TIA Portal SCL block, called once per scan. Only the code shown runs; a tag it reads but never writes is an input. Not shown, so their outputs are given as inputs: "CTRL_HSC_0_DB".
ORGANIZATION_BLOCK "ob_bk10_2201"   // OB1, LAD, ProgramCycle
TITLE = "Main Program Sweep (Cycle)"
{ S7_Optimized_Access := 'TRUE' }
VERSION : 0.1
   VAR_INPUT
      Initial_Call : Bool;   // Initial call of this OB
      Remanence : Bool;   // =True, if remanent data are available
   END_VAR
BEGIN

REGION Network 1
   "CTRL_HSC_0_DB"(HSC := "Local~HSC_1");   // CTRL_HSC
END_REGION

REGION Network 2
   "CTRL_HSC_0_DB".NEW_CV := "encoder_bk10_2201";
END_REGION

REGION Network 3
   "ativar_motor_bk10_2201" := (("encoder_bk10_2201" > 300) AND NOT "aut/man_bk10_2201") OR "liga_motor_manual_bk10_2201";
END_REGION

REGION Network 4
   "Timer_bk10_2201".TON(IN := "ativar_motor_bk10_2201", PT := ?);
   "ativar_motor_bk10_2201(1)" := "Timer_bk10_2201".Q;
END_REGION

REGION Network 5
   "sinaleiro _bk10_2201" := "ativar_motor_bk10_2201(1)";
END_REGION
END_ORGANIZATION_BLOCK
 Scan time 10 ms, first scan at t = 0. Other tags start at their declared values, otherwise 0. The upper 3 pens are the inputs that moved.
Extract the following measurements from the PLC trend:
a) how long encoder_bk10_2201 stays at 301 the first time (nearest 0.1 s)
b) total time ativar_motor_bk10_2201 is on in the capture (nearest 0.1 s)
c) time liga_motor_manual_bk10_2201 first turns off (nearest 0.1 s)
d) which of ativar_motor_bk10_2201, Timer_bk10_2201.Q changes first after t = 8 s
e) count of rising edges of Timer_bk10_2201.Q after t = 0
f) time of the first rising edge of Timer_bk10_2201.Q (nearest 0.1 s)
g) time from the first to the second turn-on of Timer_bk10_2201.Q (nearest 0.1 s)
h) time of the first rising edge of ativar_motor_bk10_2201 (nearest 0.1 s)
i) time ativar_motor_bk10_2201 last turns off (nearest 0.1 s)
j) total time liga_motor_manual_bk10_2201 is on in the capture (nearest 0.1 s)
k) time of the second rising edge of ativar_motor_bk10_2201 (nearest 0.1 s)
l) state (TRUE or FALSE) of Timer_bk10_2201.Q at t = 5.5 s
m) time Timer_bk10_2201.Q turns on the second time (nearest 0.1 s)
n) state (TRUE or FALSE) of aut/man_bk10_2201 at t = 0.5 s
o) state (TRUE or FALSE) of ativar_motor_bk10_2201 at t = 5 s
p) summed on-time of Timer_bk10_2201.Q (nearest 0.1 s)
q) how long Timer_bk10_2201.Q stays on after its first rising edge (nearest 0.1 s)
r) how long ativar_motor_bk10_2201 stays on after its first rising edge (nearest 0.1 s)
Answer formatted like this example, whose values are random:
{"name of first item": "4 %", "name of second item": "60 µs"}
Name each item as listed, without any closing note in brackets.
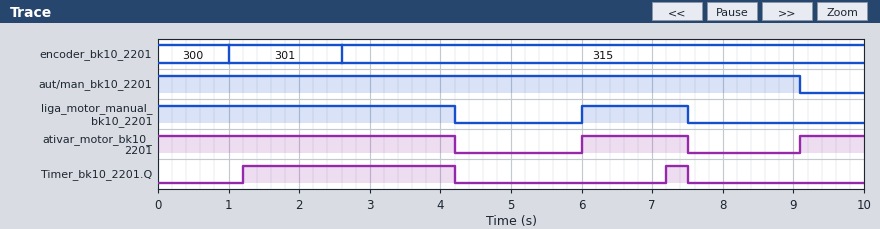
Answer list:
{"how long encoder_bk10_2201 stays at 301 the first time": "1.6 s", "total time ativar_motor_bk10_2201 is on in the capture": "6.6 s", "time liga_motor_manual_bk10_2201 first turns off": "4.2 s", "which of ativar_motor_bk10_2201, Timer_bk10_2201.Q changes first after t = 8 s": "ativar_motor_bk10_2201", "count of rising edges of Timer_bk10_2201.Q after t = 0": "2", "time of the first rising edge of Timer_bk10_2201.Q": "1.2 s", "time from the first to the second turn-on of Timer_bk10_2201.Q": "6.0 s", "time of the first rising edge of ativar_motor_bk10_2201": "6.0 s", "time ativar_motor_bk10_2201 last turns off": "7.5 s", "total time liga_motor_manual_bk10_2201 is on in the capture": "5.7 s", "time of the second rising edge of ativar_motor_bk10_2201": "9.1 s", "state (TRUE or FALSE) of Timer_bk10_2201.Q at t = 5.5 s": "FALSE", "time Timer_bk10_2201.Q turns on the second time": "7.2 s", "state (TRUE or FALSE) of aut/man_bk10_2201 at t = 0.5 s": "TRUE", "state (TRUE or FALSE) of ativar_motor_bk10_2201 at t = 5 s": "FALSE", "summed on-time of Timer_bk10_2201.Q": "3.3 s", "how long Timer_bk10_2201.Q stays on after its first rising edge": "3.0 s", "how long ativar_motor_bk10_2201 stays on after its first rising edge": "1.5 s"}
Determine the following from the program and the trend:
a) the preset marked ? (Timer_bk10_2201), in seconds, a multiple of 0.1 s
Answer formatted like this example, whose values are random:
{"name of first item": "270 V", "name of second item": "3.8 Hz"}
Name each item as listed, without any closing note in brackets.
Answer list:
{"the preset marked ? (Timer_bk10_2201), in seconds, a multiple of 0.1 s": "1.2 s"}
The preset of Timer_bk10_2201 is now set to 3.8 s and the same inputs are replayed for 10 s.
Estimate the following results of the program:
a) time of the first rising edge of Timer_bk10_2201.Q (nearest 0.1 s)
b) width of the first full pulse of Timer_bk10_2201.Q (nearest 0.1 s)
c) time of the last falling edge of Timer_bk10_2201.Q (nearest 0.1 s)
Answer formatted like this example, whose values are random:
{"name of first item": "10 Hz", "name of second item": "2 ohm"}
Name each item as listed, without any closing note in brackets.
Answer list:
{"time of the first rising edge of Timer_bk10_2201.Q": "3.8 s", "width of the first full pulse of Timer_bk10_2201.Q": "0.4 s", "time of the last falling edge of Timer_bk10_2201.Q": "4.2 s"}
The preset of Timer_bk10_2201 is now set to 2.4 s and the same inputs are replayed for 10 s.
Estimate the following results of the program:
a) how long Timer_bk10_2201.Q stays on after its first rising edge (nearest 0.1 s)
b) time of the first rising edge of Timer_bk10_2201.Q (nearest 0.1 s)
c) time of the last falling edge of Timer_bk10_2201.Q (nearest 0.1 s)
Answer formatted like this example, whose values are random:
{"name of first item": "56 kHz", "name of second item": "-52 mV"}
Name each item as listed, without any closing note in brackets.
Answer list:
{"how long Timer_bk10_2201.Q stays on after its first rising edge": "1.8 s", "time of the first rising edge of Timer_bk10_2201.Q": "2.4 s", "time of the last falling edge of Timer_bk10_2201.Q": "4.2 s"}
